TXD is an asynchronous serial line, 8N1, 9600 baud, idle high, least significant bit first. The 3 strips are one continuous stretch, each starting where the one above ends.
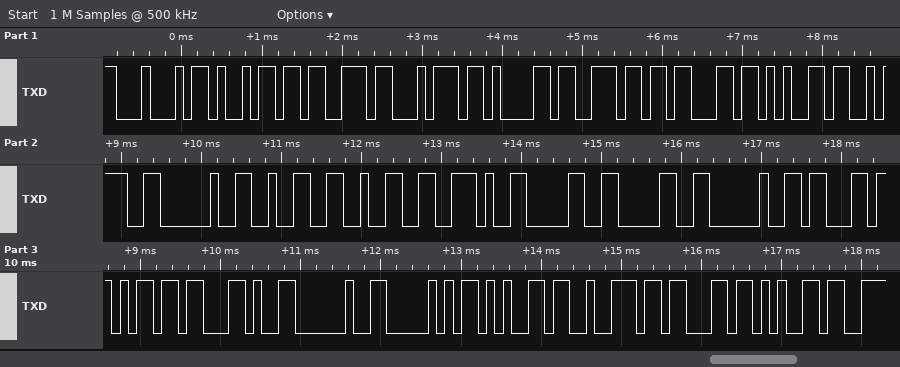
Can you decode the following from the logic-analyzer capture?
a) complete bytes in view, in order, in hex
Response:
44 69 73 74 61 6E 63 65 3A 20 32 32 2E 30 30 20 63 6D 2C 20 50 65 72 63 65
